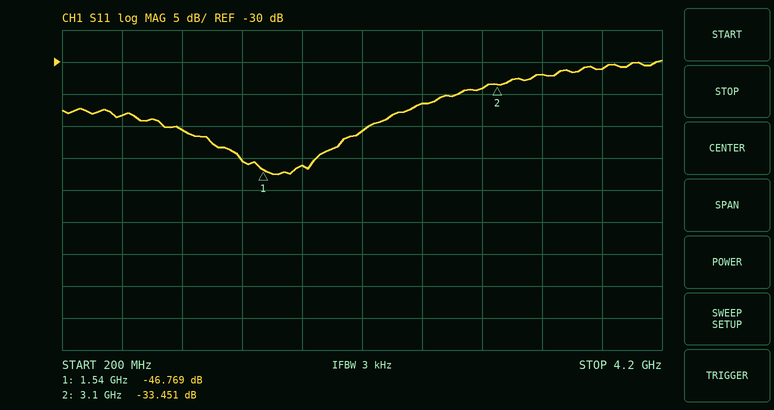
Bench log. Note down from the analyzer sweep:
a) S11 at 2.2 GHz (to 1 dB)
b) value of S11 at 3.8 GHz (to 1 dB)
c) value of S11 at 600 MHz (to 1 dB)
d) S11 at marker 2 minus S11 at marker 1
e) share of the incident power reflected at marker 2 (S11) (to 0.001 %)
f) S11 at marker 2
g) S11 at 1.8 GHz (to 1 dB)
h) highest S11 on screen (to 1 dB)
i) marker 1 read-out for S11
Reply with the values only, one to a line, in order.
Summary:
-41 dB
-31 dB
-38 dB
13.318 dB
0.045 %
-33.451 dB
-46 dB
-30 dB
-46.769 dB
